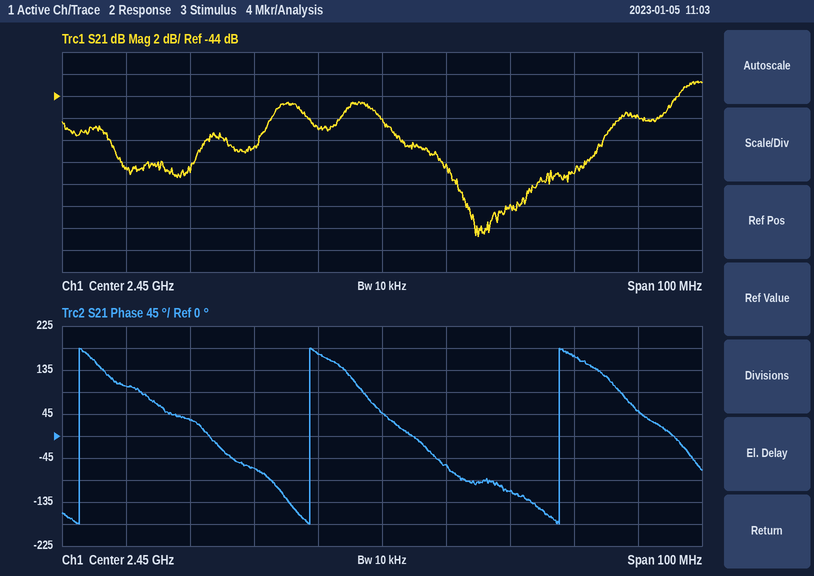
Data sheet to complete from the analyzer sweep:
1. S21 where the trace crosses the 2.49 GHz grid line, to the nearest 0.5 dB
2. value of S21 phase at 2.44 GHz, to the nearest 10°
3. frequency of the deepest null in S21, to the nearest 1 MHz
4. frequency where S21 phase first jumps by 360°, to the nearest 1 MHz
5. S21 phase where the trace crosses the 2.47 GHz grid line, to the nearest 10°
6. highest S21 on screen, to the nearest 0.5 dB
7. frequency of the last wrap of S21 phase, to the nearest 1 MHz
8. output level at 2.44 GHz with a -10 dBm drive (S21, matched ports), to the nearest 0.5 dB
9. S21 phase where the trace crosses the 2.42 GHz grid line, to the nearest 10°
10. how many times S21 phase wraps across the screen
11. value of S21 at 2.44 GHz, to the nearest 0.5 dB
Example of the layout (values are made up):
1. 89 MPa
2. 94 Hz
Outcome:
1. -46.0 dB
2. 170°
3. 2.465 GHz
4. 2.403 GHz
5. -110°
6. -42.5 dB
7. 2.478 GHz
8. -57.0 dBm
9. 30°
10. 3
11. -47.0 dB
